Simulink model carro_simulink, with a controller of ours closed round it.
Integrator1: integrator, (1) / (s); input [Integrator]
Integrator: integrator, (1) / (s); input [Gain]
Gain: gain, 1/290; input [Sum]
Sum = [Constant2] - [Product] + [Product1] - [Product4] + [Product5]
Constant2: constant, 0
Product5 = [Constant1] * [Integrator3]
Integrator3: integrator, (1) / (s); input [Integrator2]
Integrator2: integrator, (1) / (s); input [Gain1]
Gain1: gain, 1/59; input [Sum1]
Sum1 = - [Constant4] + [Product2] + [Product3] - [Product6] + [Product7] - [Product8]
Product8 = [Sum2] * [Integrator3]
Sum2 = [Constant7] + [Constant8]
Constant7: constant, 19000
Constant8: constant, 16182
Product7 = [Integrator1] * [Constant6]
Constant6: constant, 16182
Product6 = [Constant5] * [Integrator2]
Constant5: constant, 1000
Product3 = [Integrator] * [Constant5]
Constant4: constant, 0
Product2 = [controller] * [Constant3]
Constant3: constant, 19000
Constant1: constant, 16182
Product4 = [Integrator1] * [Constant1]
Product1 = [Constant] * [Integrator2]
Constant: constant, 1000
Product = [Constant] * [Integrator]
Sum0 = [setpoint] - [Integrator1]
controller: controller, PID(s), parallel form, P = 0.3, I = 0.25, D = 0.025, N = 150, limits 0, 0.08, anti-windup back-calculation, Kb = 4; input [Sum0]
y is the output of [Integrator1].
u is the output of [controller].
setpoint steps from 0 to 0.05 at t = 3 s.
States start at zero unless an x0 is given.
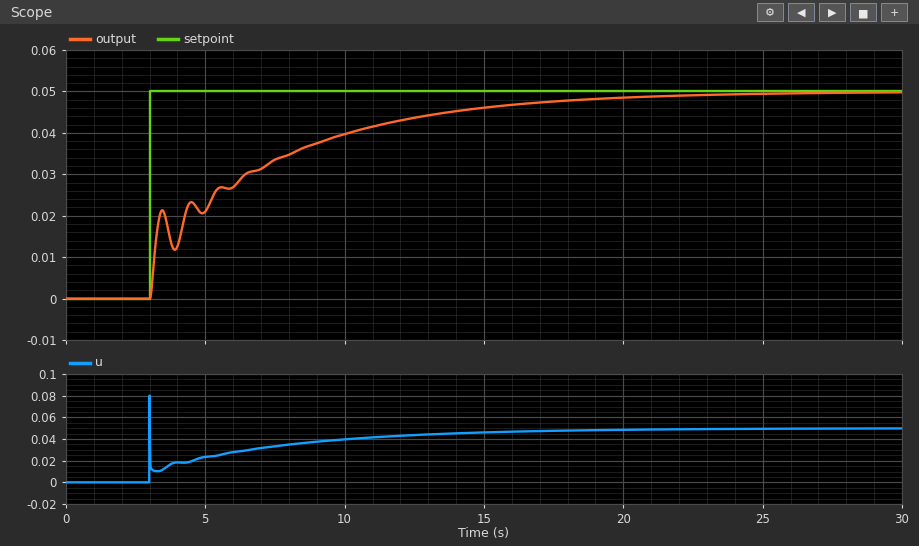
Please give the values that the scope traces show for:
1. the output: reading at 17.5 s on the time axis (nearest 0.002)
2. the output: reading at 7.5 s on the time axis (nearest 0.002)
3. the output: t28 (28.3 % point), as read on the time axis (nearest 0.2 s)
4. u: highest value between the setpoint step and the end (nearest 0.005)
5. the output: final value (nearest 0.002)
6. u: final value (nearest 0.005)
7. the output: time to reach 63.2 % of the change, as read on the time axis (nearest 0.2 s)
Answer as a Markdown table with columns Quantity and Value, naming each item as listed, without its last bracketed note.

| Quantity | Value |
|---|---|
| the output: reading at 17.5 s on the time axis | 0.048 |
| the output: reading at 7.5 s on the time axis | 0.034 |
| the output: t28 (28.3 % point), as read on the time axis | 3.2 s |
| u: highest value between the setpoint step and the end | 0.080 |
| the output: final value | 0.050 |
| u: final value | 0.050 |
| the output: time to reach 63.2 % of the change, as read on the time axis | 7.0 s |
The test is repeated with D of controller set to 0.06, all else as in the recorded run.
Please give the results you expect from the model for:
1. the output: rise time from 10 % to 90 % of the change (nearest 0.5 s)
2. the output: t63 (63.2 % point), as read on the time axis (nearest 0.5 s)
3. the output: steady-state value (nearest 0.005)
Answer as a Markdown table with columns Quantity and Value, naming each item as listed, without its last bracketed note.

| Quantity | Value |
|---|---|
| the output: rise time from 10 % to 90 % of the change | 11.0 s |
| the output: t63 (63.2 % point), as read on the time axis | 7.5 s |
| the output: steady-state value | 0.050 |
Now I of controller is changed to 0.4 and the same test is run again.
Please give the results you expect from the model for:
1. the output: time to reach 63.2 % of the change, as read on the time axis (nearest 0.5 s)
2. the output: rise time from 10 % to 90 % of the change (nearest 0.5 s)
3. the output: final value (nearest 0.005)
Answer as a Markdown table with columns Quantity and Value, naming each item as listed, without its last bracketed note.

| Quantity | Value |
|---|---|
| the output: time to reach 63.2 % of the change, as read on the time axis | 5.5 s |
| the output: rise time from 10 % to 90 % of the change | 6.5 s |
| the output: final value | 0.050 |
